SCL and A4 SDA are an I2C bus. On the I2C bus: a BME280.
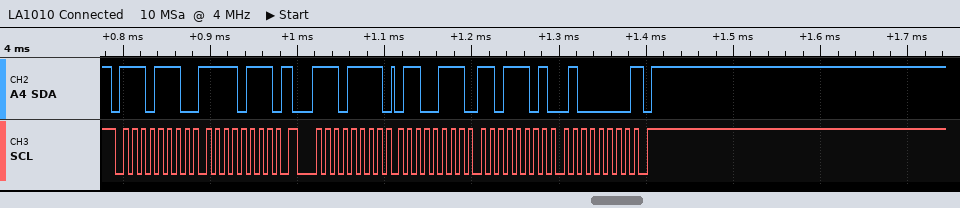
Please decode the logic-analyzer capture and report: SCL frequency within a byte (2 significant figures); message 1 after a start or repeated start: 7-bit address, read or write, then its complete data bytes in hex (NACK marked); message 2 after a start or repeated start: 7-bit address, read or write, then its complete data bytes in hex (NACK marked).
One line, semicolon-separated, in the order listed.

100 kHz; 0x77 write: F7; 0x77 read: 67 DD 40 NACK
